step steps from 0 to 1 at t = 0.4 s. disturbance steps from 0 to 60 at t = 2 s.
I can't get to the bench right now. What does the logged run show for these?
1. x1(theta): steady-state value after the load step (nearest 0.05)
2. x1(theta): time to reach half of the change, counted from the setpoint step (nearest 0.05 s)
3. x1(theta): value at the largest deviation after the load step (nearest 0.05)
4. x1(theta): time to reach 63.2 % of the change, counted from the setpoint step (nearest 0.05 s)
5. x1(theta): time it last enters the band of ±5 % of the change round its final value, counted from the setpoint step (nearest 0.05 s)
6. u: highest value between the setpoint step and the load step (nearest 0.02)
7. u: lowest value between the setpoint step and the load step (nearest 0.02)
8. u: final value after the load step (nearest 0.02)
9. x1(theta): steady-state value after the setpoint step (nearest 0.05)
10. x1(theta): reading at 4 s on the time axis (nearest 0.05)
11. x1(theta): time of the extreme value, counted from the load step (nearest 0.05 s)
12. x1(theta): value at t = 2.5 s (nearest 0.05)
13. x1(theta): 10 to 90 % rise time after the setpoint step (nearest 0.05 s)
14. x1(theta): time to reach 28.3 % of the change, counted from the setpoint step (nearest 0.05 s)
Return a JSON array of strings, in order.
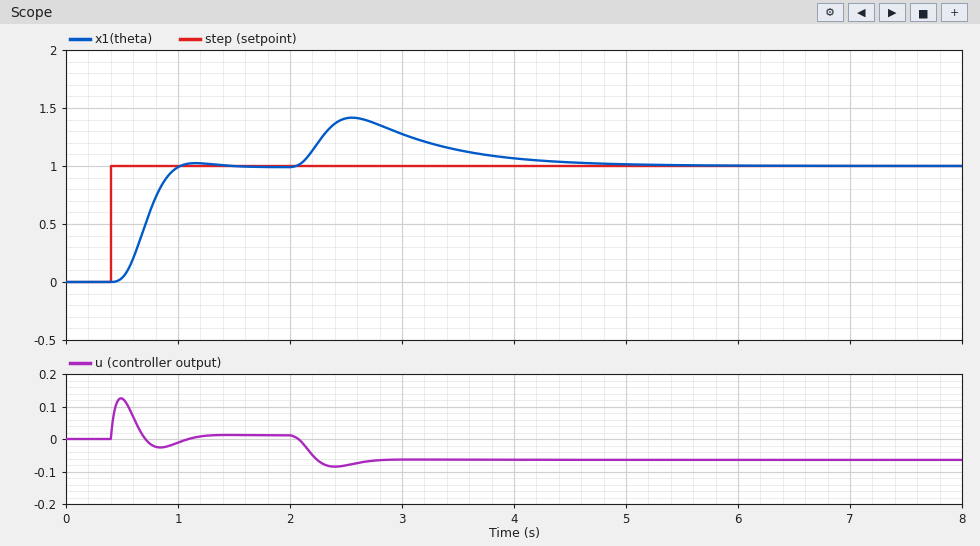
["1.00", "0.30 s", "1.40", "0.35 s", "0.55 s", "0.12", "-0.02", "-0.06", "1.00", "1.05", "0.55 s", "1.40", "0.35 s", "0.25 s"]
